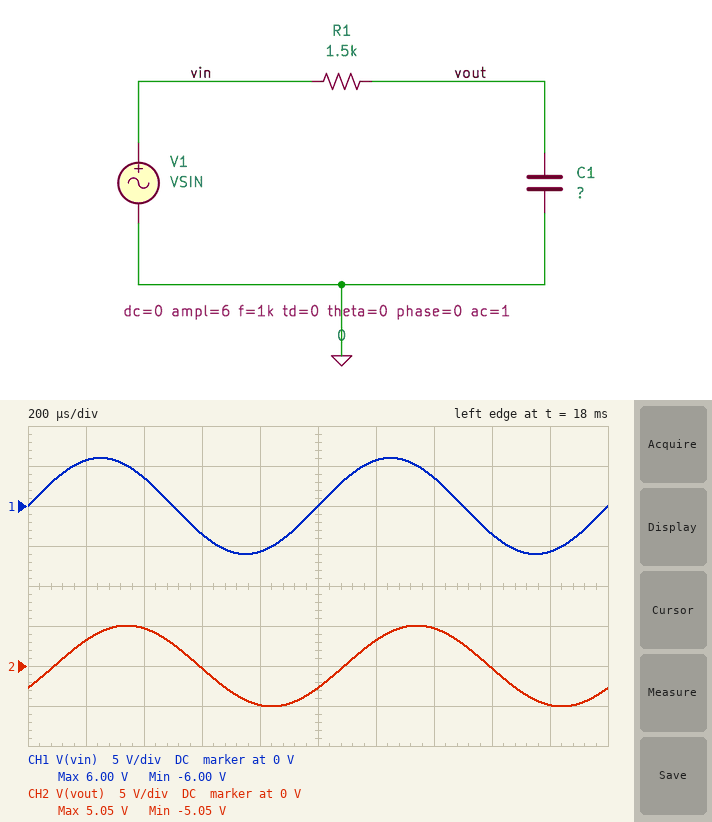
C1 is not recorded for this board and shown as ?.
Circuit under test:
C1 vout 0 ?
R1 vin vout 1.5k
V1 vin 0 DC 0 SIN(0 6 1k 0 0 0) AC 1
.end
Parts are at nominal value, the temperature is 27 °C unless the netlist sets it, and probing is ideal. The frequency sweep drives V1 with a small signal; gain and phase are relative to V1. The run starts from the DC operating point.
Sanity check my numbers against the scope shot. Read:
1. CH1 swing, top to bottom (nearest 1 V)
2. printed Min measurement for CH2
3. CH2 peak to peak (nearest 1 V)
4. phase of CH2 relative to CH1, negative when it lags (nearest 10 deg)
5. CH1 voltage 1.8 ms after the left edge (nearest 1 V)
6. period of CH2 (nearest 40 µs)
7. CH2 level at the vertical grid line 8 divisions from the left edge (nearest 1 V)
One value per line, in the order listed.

12 V
-5.05 V
10 V
-30 deg
-6 V
1.00 ms
0 V
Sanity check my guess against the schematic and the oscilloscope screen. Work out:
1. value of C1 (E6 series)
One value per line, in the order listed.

68 nF
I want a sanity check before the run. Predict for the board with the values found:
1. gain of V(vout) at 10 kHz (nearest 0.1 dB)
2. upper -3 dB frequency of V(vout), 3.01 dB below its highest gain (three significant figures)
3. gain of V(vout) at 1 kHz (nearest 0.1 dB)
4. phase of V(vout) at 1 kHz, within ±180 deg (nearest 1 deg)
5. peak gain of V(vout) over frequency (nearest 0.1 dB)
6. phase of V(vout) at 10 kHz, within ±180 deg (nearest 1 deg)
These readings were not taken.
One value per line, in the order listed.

-16.2 dB
1.56 kHz
-1.5 dB
-33 deg
0 dB
-81 deg
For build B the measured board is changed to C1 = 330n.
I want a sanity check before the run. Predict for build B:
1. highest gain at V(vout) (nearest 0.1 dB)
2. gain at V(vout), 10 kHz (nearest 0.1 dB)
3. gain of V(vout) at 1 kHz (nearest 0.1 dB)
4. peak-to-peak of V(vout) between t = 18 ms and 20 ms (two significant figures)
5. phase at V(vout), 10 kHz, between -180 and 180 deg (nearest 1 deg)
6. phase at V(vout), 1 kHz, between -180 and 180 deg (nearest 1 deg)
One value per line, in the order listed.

0 dB
-29.9 dB
-10.3 dB
3.7 V
-88 deg
-72 deg
